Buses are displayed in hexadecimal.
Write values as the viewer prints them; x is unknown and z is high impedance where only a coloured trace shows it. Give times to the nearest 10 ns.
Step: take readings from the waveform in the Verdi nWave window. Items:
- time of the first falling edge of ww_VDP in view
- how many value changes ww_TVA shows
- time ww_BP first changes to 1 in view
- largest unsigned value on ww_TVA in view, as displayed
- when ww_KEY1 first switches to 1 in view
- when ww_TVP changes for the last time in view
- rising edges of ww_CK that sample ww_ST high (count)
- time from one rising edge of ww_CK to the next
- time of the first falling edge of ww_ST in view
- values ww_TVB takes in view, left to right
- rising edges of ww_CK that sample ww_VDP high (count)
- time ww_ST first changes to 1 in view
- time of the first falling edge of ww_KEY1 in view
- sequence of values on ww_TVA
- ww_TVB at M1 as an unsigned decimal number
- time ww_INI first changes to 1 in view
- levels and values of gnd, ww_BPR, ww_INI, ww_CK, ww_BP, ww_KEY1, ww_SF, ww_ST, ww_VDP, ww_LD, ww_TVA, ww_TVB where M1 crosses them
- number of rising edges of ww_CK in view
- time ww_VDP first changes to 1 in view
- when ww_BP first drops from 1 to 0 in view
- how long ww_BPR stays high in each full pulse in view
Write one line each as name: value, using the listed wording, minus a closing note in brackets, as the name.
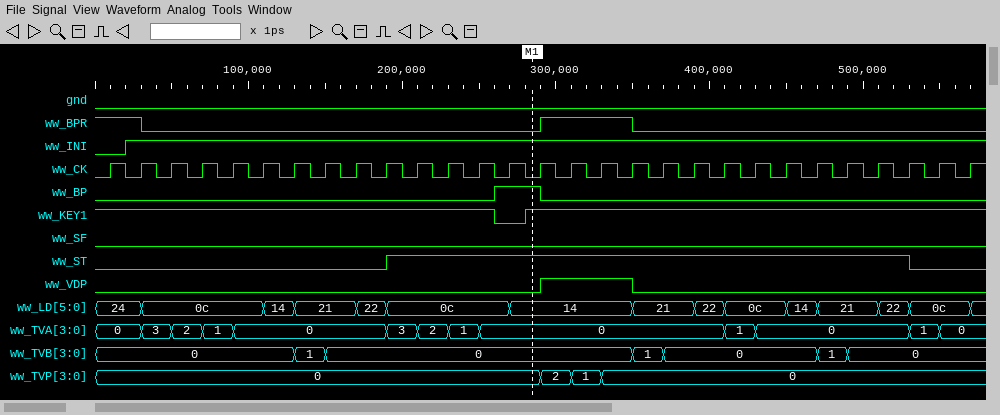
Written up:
time of the first falling edge of ww_VDP in view: 350 ns
how many value changes ww_TVA shows: 12
time ww_BP first changes to 1 in view: 260 ns
largest unsigned value on ww_TVA in view, as displayed: 3
when ww_KEY1 first switches to 1 in view: 280 ns
when ww_TVP changes for the last time in view: 330 ns
rising edges of ww_CK that sample ww_ST high: 17
time from one rising edge of ww_CK to the next: 20 ns
time of the first falling edge of ww_ST in view: 530 ns
values ww_TVB takes in view, left to right: 0, 1, 0, 1, 0, 1, 0
rising edges of ww_CK that sample ww_VDP high: 3
time ww_ST first changes to 1 in view: 190 ns
time of the first falling edge of ww_KEY1 in view: 260 ns
sequence of values on ww_TVA: 0, 3, 2, 1, 0, 3, 2, 1, 0, 1, 0, 1, 0
ww_TVB at M1 as an unsigned decimal number: 0
time ww_INI first changes to 1 in view: 20 ns
levels and values of gnd, ww_BPR, ww_INI, ww_CK, ww_BP, ww_KEY1, ww_SF, ww_ST, ww_VDP, ww_LD, ww_TVA, ww_TVB where M1 crosses them: gnd=0, ww_BPR=0, ww_INI=1, ww_CK=0, ww_BP=1, ww_KEY1=1, ww_SF=0, ww_ST=1, ww_VDP=0, ww_LD=14, ww_TVA=0, ww_TVB=0
number of rising edges of ww_CK in view: 29
time ww_VDP first changes to 1 in view: 290 ns
when ww_BP first drops from 1 to 0 in view: 290 ns
how long ww_BPR stays high in each full pulse in view: 60 ns
